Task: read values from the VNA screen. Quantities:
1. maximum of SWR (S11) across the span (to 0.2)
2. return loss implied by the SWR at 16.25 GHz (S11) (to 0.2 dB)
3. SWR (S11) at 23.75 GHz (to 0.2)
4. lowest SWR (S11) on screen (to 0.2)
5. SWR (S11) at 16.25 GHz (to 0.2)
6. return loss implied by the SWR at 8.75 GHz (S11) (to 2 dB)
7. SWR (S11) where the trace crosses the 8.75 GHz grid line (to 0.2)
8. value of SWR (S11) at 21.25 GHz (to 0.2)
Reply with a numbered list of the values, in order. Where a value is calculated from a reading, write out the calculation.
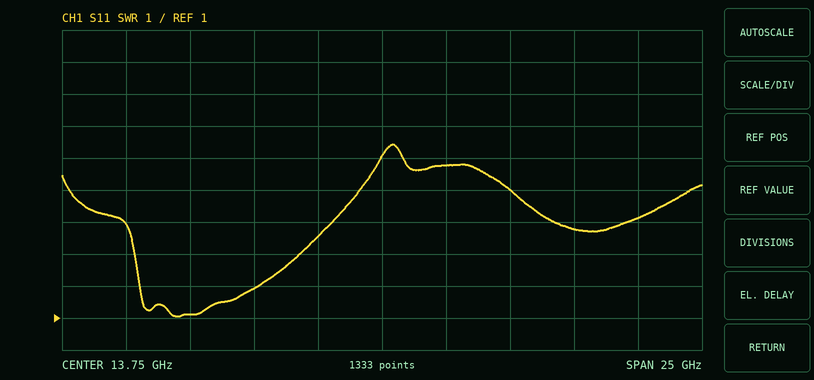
1. 6.4
2. −20 log10((5.8 − 1)/(5.8 + 1)) ≈ 3.0 dB
3. 4.2
4. 1.0
5. 5.8
6. −20 log10((2 − 1)/(2 + 1)) ≈ 10 dB
7. 2.0
8. 3.8
